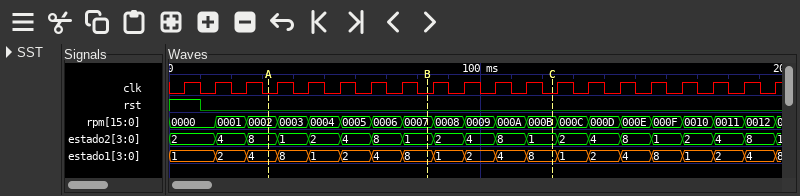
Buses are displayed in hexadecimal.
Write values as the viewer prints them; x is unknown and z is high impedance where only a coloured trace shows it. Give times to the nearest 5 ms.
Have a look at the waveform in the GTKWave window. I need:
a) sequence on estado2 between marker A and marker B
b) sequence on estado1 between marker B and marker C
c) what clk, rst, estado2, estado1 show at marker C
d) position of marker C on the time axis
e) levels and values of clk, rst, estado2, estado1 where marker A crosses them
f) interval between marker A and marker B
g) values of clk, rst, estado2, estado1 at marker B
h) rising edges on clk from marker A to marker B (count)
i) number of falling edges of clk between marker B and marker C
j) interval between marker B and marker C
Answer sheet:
8, 1, 2, 4, 8, 1
8, 1, 2, 4, 8
clk=0, rst=0, estado2=1, estado1=8
125 ms
clk=0, rst=0, estado2=8, estado1=4
50 ms
clk=0, rst=0, estado2=1, estado1=8
5
4
40 ms
